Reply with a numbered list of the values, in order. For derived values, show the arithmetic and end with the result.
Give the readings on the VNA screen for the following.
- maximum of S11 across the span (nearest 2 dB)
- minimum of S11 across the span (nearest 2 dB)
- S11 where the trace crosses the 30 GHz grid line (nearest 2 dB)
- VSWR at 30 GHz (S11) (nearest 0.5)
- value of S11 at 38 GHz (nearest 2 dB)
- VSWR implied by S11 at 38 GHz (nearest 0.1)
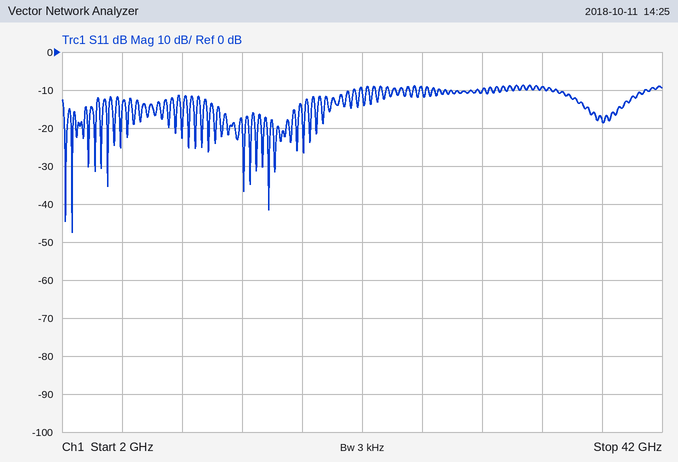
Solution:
1. -8 dB
2. -48 dB
3. -10 dB
4. |Γ| = 10^(-10/20) = 0.3162; VSWR = (1 + 0.3162)/(1 − 0.3162) ≈ 1.92, so 2.0 to the nearest 0.5
5. -18 dB
6. |Γ| = 10^(-18/20) = 0.1259; VSWR = (1 + 0.1259)/(1 − 0.1259) ≈ 1.3
